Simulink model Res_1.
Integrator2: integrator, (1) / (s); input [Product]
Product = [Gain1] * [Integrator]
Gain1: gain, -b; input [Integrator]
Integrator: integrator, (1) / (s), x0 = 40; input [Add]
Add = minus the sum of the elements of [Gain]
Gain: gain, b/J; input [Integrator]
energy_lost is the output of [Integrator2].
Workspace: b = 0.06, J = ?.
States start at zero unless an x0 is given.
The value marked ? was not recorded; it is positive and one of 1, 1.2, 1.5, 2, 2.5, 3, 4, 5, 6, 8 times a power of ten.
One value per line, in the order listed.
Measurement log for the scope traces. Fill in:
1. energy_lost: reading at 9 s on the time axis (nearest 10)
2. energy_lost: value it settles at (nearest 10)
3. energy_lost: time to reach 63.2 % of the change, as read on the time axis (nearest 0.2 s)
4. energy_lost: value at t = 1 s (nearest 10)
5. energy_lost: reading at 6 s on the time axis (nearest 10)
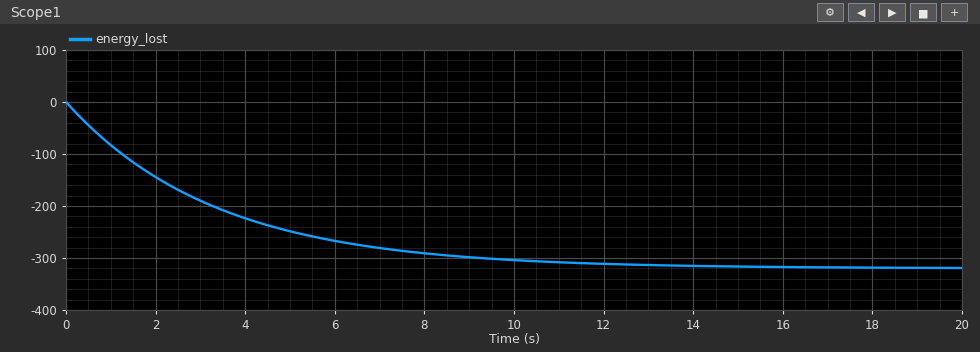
-300
-320
3.4 s
-80
-270
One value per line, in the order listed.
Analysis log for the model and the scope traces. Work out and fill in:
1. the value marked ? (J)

0.4
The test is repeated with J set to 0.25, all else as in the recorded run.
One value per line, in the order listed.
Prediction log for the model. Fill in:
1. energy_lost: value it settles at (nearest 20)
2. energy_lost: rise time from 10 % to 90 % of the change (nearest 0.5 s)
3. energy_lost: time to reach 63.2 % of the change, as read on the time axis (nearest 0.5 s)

-200
4.5 s
2.0 s
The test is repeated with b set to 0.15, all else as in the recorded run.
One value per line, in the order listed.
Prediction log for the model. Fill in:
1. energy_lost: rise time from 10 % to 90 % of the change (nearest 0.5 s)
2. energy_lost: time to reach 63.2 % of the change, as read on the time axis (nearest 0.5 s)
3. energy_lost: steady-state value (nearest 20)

3.0 s
1.5 s
-320
